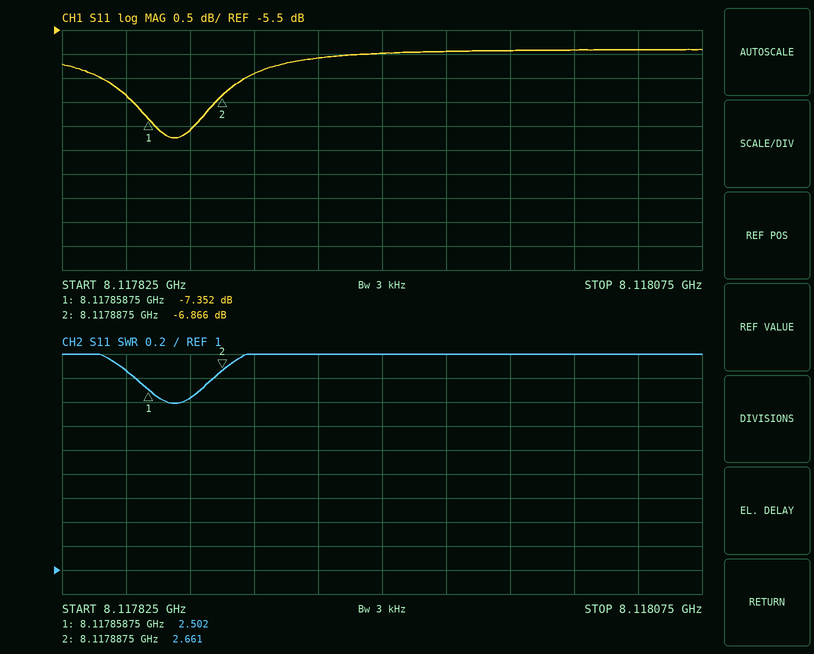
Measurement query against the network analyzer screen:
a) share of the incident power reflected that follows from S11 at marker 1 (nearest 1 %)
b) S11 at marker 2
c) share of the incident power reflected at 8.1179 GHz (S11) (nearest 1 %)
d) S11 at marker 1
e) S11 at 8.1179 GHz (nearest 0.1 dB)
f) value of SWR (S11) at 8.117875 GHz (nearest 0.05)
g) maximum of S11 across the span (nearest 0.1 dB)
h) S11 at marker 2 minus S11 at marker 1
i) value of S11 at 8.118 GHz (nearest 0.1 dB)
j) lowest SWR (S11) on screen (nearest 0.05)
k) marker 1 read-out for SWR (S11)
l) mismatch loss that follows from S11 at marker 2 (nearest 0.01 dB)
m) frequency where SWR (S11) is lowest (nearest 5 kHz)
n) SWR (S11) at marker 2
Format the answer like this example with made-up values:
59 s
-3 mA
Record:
18 %
-6.866 dB
23 %
-7.352 dB
-6.4 dB
2.45
-5.9 dB
0.486 dB
-5.9 dB
2.40
2.502
1.00 dB
8.117870 GHz
2.661
